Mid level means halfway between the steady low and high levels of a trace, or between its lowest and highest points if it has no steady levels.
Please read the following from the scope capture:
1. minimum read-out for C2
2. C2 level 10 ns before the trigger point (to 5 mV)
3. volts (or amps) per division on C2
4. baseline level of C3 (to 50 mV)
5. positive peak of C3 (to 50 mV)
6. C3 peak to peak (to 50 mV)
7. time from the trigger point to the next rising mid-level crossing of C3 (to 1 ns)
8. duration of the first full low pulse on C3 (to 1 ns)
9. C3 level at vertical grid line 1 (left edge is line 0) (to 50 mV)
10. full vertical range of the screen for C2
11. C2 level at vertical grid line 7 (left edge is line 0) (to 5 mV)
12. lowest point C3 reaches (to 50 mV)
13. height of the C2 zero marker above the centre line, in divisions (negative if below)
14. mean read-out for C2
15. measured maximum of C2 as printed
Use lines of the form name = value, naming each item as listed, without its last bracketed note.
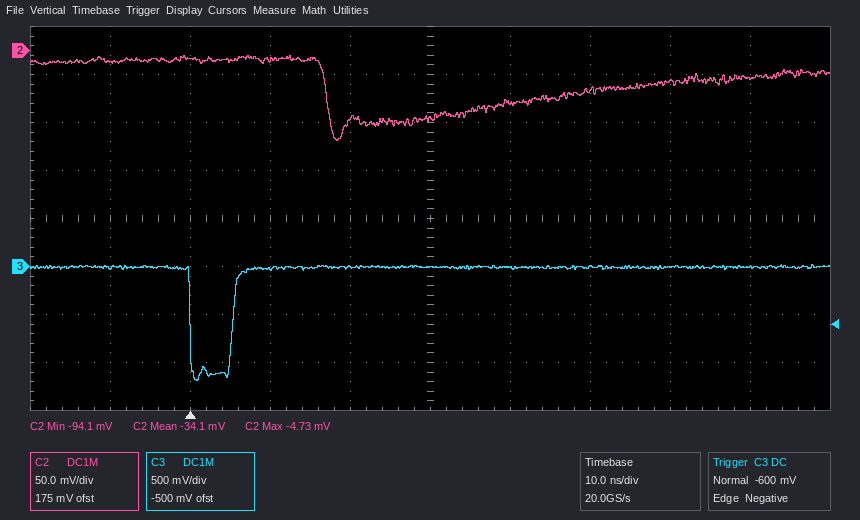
minimum read-out for C2 = -94.1 mV
C2 level 10 ns before the trigger point = -10 mV
volts (or amps) per division on C2 = 50 mV
baseline level of C3 = 0 mV
positive peak of C3 = 0 mV
C3 peak to peak = 1.20 V
time from the trigger point to the next rising mid-level crossing of C3 = 5 ns
duration of the first full low pulse on C3 = 5 ns
C3 level at vertical grid line 1 (left edge is line 0) = 0 mV
full vertical range of the screen for C2 = 400 mV
C2 level at vertical grid line 7 (left edge is line 0) = -40 mV
lowest point C3 reaches = -1.20 V
height of the C2 zero marker above the centre line, in divisions = +3.5 div
mean read-out for C2 = -34.1 mV
measured maximum of C2 as printed = -4.73 mV
